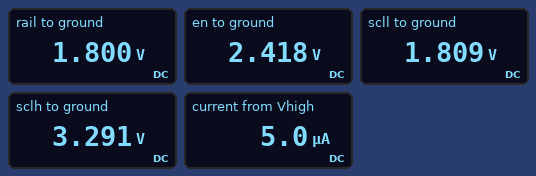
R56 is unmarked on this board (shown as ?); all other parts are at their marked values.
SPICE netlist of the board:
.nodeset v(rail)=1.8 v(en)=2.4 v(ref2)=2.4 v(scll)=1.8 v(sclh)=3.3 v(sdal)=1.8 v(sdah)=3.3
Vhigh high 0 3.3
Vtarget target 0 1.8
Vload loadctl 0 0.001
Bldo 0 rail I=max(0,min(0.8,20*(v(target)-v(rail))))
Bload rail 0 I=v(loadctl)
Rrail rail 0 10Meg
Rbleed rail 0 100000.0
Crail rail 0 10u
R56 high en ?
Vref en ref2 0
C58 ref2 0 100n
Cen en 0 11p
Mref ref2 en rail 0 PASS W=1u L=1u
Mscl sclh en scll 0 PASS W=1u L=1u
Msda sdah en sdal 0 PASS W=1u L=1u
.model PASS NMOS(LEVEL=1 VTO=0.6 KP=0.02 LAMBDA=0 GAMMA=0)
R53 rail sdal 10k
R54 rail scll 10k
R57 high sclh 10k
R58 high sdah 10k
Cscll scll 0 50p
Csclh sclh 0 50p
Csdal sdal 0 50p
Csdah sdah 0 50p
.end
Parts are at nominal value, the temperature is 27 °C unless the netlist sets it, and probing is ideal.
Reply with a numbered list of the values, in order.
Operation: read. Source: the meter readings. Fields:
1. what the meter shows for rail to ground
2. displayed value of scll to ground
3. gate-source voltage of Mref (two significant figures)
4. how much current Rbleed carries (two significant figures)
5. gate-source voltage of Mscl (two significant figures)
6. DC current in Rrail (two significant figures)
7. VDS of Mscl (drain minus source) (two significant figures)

1. 1.800 V
2. 1.809 V
3. 620 mV
4. 18 µA
5. 610 mV
6. 180 nA
7. 1.5 V
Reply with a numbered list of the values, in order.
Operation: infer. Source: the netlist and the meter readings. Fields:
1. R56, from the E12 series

1. 270 kΩ
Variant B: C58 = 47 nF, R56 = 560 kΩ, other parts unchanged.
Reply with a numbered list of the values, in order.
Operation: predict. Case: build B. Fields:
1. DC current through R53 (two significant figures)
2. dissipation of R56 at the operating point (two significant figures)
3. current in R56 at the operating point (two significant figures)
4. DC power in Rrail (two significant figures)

1. 530 nA
2. 1.4 µW
3. 1.6 µA
4. 320 nW
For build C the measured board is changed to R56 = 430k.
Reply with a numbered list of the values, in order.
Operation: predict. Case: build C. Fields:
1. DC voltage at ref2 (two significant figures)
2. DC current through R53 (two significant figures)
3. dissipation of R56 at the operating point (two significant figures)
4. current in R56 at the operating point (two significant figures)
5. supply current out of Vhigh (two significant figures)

1. 2.4 V
2. 640 nA
3. 1.8 µW
4. 2.1 µA
5. 3.3 µA
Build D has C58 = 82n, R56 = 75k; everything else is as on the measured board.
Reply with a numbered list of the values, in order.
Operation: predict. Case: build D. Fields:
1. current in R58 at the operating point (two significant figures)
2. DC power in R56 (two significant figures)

1. 2.0 µA
2. 10 µW
